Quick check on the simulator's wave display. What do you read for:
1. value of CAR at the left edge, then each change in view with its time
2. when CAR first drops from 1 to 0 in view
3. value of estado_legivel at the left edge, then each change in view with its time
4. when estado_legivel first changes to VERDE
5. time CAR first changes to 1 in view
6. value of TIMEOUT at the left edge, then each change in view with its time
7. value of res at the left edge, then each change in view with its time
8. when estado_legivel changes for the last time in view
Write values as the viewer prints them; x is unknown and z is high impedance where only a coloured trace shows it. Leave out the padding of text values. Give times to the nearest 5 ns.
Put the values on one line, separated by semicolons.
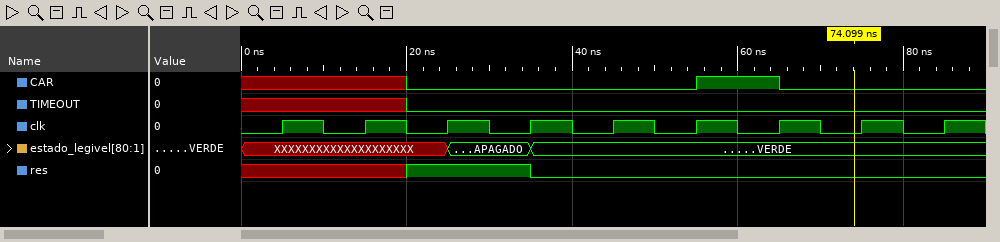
x, 0 at 20 ns, 1 at 55 ns, 0 at 65 ns; 65 ns; XXXXXXXXXXXXXXXXXXXX, APAGADO at 25 ns, VERDE at 35 ns; 35 ns; 55 ns; x, 0 at 20 ns; x, 1 at 20 ns, 0 at 35 ns; 35 ns
